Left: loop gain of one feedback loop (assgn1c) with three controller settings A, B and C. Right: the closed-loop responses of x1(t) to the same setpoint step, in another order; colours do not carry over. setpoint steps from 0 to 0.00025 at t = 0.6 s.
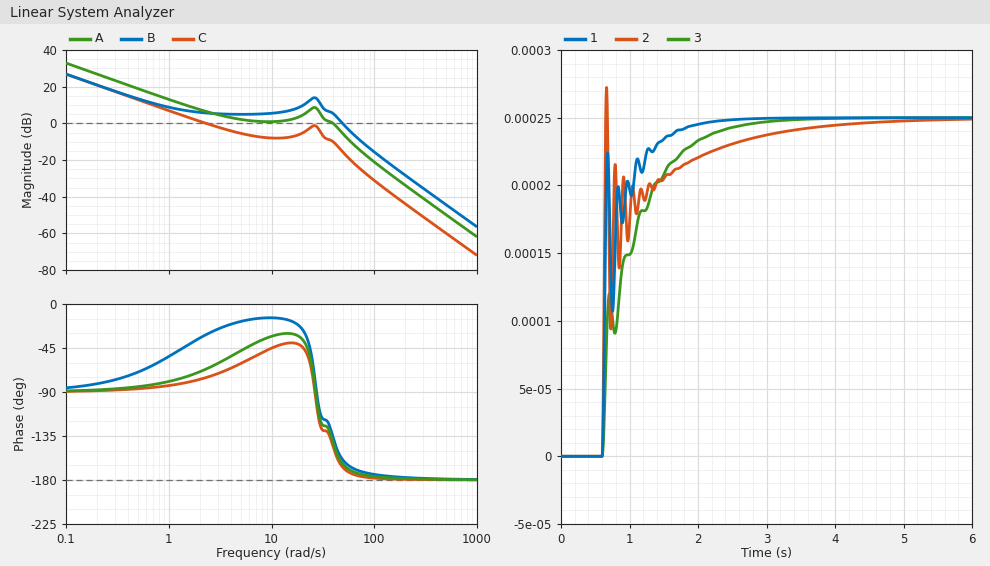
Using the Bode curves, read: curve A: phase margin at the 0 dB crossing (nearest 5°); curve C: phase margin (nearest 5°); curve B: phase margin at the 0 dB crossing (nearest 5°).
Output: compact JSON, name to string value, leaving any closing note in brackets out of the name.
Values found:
{"curve A: phase margin at the 0 dB crossing": "40°", "curve C: phase margin": "105°", "curve B: phase margin at the 0 dB crossing": "20°"}
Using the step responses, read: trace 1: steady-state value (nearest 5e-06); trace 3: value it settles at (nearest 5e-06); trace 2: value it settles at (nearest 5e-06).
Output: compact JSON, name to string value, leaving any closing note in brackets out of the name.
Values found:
{"trace 1: steady-state value": "0.000250", "trace 3: value it settles at": "0.000250", "trace 2: value it settles at": "0.000250"}
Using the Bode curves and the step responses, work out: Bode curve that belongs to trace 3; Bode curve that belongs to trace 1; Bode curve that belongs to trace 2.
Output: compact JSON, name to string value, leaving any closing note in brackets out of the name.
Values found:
{"Bode curve that belongs to trace 3": "C", "Bode curve that belongs to trace 1": "A", "Bode curve that belongs to trace 2": "B"}
